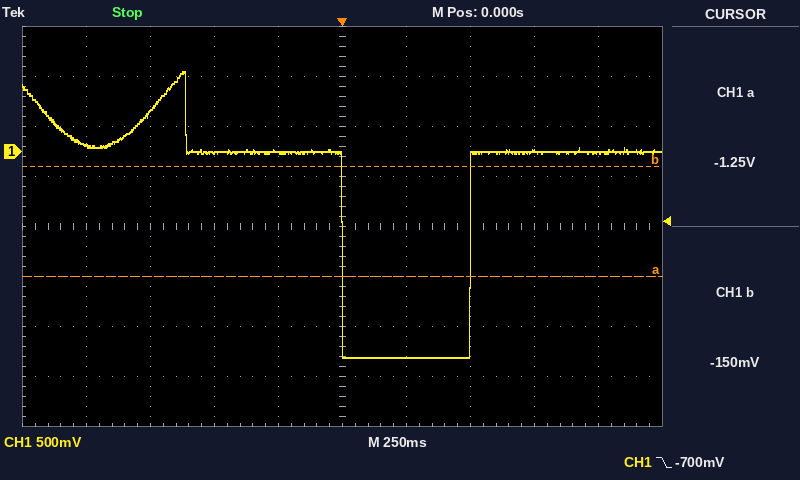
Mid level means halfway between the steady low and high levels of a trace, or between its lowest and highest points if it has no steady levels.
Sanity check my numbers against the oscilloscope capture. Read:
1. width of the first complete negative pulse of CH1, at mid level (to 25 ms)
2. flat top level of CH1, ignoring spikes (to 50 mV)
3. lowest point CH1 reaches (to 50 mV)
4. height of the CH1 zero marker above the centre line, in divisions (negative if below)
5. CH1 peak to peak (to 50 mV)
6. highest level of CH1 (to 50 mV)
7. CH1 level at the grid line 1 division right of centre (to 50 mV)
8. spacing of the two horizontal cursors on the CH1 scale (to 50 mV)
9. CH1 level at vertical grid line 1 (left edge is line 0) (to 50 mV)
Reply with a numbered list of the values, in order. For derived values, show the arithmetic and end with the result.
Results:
1. 500 ms
2. 0 mV
3. -2.05 V
4. +1.5 div
5. 800 mV − (-2.05 V) = 2.85 V
6. 800 mV
7. -2.05 V
8. 1.10 V
9. 50 mV
